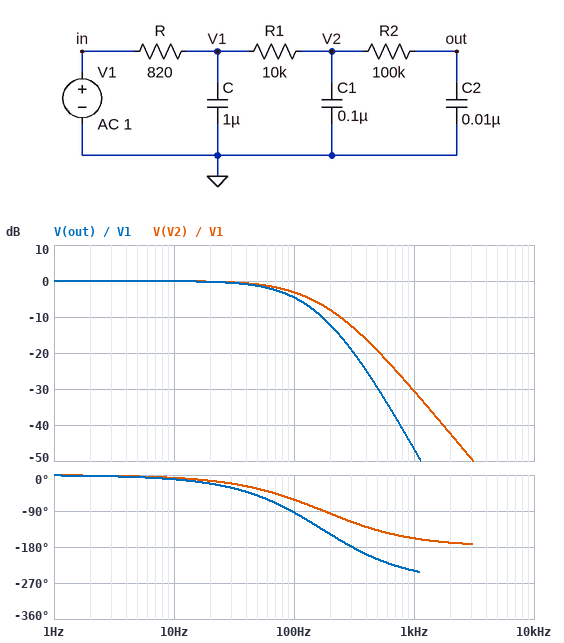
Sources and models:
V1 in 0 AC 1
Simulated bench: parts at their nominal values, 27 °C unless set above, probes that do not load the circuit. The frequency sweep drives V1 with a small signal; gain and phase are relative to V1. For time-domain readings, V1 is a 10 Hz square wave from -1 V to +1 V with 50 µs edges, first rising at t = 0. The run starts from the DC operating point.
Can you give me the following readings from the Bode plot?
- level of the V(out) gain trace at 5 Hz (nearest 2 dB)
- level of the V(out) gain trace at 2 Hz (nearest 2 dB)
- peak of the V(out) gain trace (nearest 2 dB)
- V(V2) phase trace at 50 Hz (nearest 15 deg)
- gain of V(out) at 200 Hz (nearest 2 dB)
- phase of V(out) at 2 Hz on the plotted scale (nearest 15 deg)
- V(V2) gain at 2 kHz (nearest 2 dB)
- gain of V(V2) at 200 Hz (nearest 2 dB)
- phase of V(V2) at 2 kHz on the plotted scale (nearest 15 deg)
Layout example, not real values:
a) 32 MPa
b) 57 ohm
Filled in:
a) 0 dB
b) 0 dB
c) 0 dB
d) -30 deg
e) -12 dB
f) 0 deg
g) -42 dB
h) -8 dB
i) -165 deg
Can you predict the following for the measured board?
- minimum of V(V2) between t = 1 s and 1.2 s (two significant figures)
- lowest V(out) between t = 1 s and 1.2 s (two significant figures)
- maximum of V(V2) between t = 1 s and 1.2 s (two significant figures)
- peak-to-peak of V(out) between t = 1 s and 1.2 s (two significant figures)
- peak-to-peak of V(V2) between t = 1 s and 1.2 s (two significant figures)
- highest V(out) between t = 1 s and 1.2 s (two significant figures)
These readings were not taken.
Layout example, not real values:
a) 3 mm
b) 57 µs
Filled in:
a) -1.0 V
b) -1.0 V
c) 1.0 V
d) 2.0 V
e) 2.0 V
f) 1.0 V
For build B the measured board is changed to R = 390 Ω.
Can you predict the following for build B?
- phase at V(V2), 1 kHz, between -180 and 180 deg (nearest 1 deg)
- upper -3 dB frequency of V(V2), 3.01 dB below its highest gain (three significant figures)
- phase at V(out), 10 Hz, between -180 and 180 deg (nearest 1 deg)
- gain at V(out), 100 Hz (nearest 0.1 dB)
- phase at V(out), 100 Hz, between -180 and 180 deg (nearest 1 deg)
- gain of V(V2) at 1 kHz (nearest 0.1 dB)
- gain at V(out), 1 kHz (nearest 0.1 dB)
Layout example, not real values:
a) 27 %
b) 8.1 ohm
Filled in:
a) -147 deg
b) 124 Hz
c) -9 deg
d) -3.6 dB
e) -80 deg
f) -24.6 dB
g) -40.7 dB
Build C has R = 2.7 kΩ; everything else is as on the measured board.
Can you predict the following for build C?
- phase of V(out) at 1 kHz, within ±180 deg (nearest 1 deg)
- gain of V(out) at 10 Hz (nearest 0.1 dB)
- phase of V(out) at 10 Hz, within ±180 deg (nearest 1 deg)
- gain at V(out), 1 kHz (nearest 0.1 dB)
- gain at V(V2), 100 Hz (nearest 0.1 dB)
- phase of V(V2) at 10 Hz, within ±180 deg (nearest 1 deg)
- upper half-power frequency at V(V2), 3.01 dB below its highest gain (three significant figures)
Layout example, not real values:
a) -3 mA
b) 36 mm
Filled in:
a) 113 deg
b) -0.2 dB
c) -18 deg
d) -56.8 dB
e) -8.3 dB
f) -15 deg
g) 46.2 Hz
